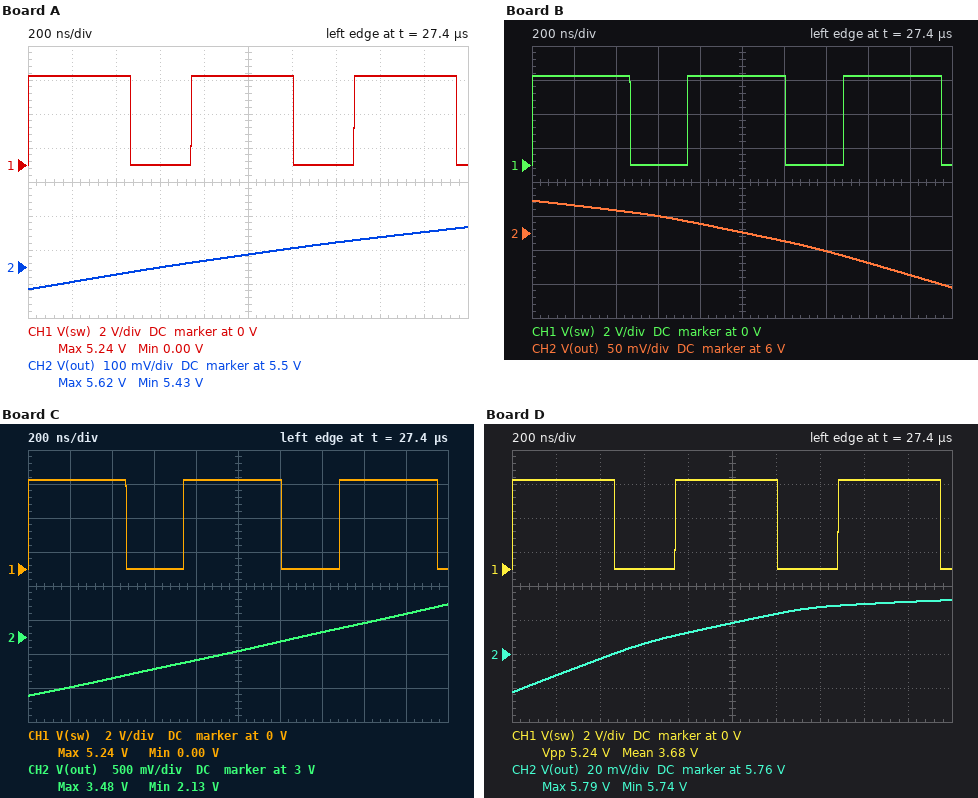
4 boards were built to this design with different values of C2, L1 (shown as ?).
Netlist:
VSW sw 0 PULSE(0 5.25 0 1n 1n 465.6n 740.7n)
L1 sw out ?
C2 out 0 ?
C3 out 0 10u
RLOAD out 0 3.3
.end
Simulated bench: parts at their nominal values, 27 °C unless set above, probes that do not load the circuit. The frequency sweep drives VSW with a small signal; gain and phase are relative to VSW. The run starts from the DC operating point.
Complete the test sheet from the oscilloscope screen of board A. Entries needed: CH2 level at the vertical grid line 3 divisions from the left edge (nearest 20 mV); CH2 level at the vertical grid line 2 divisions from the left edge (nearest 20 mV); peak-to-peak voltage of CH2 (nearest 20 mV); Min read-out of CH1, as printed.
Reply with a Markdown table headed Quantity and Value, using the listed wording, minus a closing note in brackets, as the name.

| Quantity | Value |
|---|---|
| CH2 level at the vertical grid line 3 divisions from the left edge | 5.50 V |
| CH2 level at the vertical grid line 2 divisions from the left edge | 5.48 V |
| peak-to-peak voltage of CH2 | 180 mV |
| Min read-out of CH1, as printed | 0.00 V |
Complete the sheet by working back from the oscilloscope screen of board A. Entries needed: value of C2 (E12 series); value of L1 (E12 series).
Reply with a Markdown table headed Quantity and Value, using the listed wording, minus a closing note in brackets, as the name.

| Quantity | Value |
|---|---|
| value of C2 | 5.6 µF |
| value of L1 | 6.8 µH |
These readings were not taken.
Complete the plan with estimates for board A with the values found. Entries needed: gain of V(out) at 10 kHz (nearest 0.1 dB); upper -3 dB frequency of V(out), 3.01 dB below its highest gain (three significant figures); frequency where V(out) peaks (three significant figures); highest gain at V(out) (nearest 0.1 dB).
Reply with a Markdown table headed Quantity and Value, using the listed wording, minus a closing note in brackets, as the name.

| Quantity | Value |
|---|---|
| gain of V(out) at 10 kHz | 4.5 dB |
| upper -3 dB frequency of V(out), 3.01 dB below its highest gain | 16.8 kHz |
| frequency where V(out) peaks | 15.3 kHz |
| highest gain at V(out) | 14.0 dB |
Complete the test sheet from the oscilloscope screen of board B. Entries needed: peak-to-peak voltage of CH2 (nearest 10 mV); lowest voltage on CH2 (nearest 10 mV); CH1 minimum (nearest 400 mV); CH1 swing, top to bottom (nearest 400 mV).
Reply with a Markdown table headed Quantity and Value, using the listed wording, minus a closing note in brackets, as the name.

| Quantity | Value |
|---|---|
| peak-to-peak voltage of CH2 | 130 mV |
| lowest voltage on CH2 | 5.92 V |
| CH1 minimum | 0 V |
| CH1 swing, top to bottom | 5.2 V |
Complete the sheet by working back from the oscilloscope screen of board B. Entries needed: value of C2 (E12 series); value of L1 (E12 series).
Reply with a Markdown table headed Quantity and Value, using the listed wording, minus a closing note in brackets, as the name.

| Quantity | Value |
|---|---|
| value of C2 | 12 µF |
| value of L1 | 3.3 µH |
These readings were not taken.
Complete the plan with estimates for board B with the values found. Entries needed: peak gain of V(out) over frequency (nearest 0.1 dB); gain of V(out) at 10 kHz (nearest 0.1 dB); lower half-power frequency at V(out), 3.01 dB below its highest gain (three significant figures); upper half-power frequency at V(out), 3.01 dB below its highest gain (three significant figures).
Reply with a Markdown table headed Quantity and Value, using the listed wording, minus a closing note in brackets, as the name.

| Quantity | Value |
|---|---|
| peak gain of V(out) over frequency | 18.6 dB |
| gain of V(out) at 10 kHz | 2.9 dB |
| lower half-power frequency at V(out), 3.01 dB below its highest gain | 17.5 kHz |
| upper half-power frequency at V(out), 3.01 dB below its highest gain | 19.7 kHz |
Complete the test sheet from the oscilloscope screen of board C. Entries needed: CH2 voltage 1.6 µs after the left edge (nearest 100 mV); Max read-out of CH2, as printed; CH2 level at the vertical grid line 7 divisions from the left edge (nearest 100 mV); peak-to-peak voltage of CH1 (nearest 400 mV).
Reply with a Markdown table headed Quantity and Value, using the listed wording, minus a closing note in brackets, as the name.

| Quantity | Value |
|---|---|
| CH2 voltage 1.6 µs after the left edge | 3.2 V |
| Max read-out of CH2, as printed | 3.48 V |
| CH2 level at the vertical grid line 7 divisions from the left edge | 3.1 V |
| peak-to-peak voltage of CH1 | 5.2 V |
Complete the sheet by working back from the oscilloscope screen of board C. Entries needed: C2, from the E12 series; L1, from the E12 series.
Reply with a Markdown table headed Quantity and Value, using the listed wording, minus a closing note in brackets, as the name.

| Quantity | Value |
|---|---|
| C2, from the E12 series | 6.8 µF |
| L1, from the E12 series | 820 nH |
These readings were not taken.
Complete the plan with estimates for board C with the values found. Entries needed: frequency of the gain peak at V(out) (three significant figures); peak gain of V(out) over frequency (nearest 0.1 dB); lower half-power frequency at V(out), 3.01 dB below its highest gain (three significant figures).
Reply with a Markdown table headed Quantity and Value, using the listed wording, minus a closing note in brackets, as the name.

| Quantity | Value |
|---|---|
| frequency of the gain peak at V(out) | 42.8 kHz |
| peak gain of V(out) over frequency | 23.5 dB |
| lower half-power frequency at V(out), 3.01 dB below its highest gain | 41.4 kHz |
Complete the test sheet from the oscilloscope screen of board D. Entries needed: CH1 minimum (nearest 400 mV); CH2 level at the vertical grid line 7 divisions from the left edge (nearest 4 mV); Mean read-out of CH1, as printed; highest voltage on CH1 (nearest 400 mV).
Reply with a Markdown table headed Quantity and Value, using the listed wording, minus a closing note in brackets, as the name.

| Quantity | Value |
|---|---|
| CH1 minimum | 0 V |
| CH2 level at the vertical grid line 7 divisions from the left edge | 5.788 V |
| Mean read-out of CH1, as printed | 3.68 V |
| highest voltage on CH1 | 5.2 V |
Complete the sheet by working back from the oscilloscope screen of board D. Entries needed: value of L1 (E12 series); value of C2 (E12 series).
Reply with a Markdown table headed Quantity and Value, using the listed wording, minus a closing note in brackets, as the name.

| Quantity | Value |
|---|---|
| value of L1 | 5.6 µH |
| value of C2 | 5.6 µF |
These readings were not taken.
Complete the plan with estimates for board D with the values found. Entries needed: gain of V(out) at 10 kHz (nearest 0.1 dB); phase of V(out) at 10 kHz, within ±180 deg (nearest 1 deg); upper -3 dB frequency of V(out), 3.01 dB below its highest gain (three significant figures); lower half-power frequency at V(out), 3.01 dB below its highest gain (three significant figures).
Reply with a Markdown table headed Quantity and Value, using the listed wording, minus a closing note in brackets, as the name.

| Quantity | Value |
|---|---|
| gain of V(out) at 10 kHz | 3.6 dB |
| phase of V(out) at 10 kHz, within ±180 deg | -9 deg |
| upper -3 dB frequency of V(out), 3.01 dB below its highest gain | 18.4 kHz |
| lower half-power frequency at V(out), 3.01 dB below its highest gain | 15.3 kHz |
